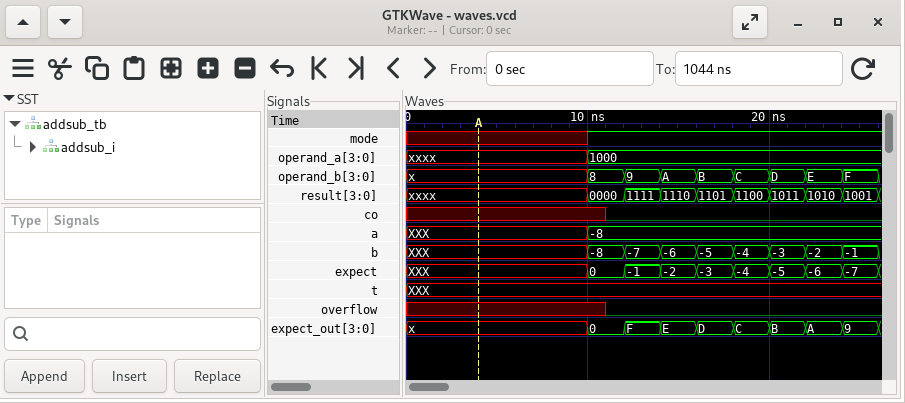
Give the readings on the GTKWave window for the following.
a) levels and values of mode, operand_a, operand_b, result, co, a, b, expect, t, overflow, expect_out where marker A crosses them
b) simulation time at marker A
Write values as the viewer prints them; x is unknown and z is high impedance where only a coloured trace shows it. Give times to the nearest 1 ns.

mode=x, operand_a=xxxx, operand_b=x, result=xxxx, co=x, a=XXX, b=XXX, expect=XXX, t=XXX, overflow=x, expect_out=x
4 ns
